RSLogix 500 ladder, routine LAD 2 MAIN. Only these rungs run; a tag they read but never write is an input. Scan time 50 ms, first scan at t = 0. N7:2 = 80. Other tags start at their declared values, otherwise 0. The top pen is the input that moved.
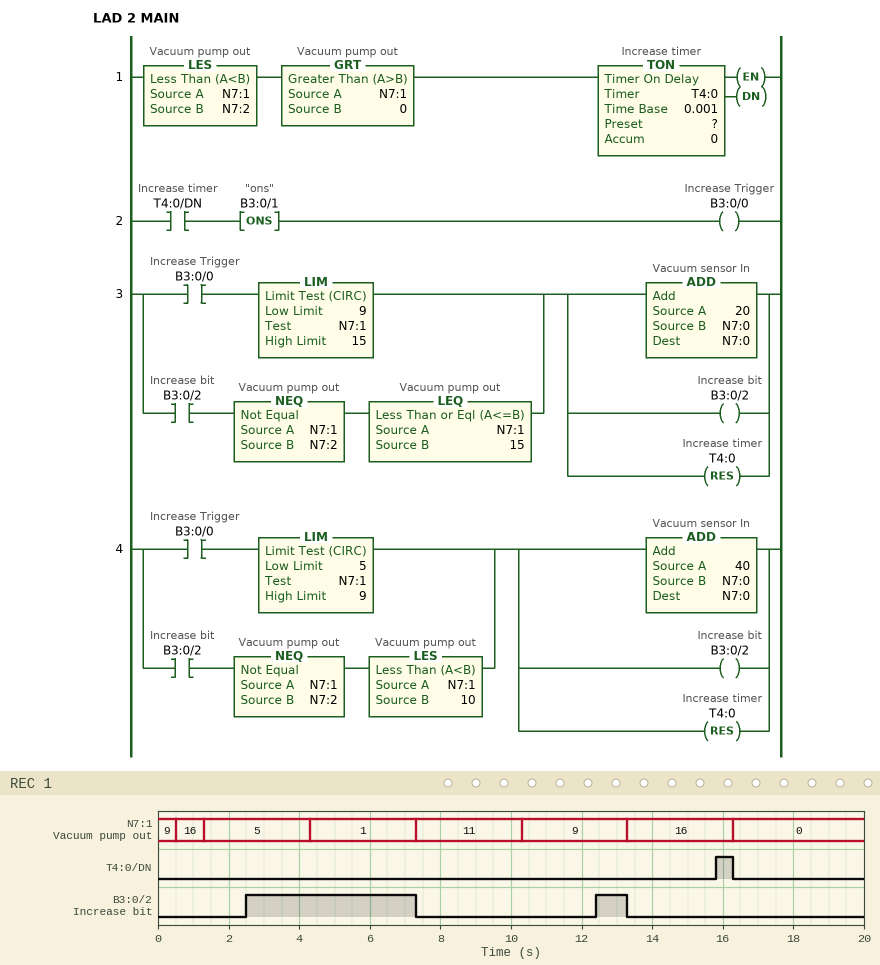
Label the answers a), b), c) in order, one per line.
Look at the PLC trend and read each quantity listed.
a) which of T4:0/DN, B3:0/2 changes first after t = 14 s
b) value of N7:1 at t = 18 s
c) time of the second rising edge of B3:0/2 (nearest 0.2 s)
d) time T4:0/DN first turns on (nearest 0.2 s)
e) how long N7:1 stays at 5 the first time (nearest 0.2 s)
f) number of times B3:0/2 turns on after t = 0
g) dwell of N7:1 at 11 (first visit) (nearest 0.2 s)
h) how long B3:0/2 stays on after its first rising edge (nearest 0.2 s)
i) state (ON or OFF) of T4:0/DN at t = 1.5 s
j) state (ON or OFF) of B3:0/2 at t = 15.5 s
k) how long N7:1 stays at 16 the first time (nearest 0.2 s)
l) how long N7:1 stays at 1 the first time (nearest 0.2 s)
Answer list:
a) T4:0/DN
b) 0
c) 12.4 s
d) 15.8 s
e) 3.0 s
f) 2
g) 3.0 s
h) 4.8 s
i) OFF
j) OFF
k) 0.8 s
l) 3.0 s
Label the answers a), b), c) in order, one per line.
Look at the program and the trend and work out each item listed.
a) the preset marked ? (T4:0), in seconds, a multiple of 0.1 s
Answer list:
a) 2.5 s
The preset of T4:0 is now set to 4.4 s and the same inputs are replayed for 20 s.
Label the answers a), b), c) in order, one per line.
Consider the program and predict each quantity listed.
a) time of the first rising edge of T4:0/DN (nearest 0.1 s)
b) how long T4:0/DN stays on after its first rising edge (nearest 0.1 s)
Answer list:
a) 4.4 s
b) 11.9 s
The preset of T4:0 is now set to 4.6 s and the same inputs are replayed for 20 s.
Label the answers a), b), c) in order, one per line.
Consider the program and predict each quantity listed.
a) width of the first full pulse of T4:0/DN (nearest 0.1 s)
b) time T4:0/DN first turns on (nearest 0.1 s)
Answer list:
a) 11.7 s
b) 4.6 s
